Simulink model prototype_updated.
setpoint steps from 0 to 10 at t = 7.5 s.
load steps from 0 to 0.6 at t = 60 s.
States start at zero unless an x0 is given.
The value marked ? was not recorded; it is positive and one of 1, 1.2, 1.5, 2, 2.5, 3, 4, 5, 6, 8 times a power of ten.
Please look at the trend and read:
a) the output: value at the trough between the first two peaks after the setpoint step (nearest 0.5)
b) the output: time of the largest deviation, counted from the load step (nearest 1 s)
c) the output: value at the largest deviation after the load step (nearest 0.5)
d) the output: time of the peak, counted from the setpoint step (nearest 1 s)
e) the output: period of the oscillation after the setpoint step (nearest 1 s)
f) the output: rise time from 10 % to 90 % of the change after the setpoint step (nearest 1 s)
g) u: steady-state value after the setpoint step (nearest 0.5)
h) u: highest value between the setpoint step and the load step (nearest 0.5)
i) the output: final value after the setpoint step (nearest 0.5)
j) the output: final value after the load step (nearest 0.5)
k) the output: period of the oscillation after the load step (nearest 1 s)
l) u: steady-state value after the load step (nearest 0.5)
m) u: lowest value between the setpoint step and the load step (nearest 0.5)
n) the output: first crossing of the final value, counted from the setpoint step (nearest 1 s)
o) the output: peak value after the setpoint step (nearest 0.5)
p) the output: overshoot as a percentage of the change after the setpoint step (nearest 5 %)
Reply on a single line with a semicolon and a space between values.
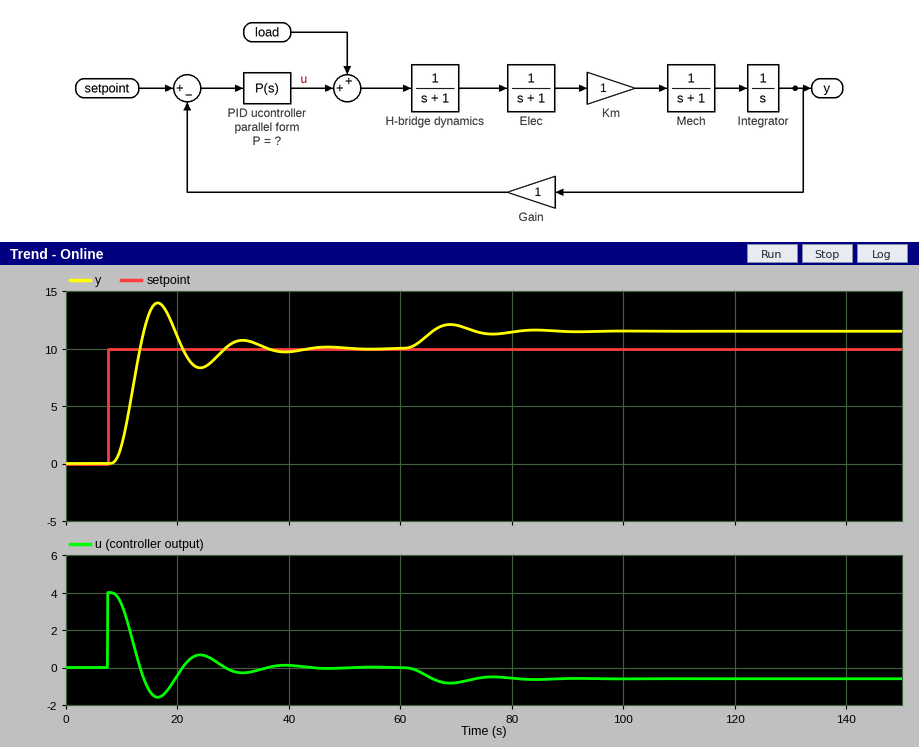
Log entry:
8.5; 9 s; 12.0; 9 s; 15 s; 3 s; 0.0; 4.0; 10.0; 11.5; 15 s; -0.5; -1.5; 6 s; 14.0; 40 %
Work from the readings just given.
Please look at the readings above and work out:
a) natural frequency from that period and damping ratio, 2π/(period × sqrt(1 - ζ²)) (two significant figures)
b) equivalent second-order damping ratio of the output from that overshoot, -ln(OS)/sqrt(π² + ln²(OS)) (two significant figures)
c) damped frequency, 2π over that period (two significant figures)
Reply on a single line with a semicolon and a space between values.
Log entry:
0.44 rad/s; 0.28; 0.42 rad/s
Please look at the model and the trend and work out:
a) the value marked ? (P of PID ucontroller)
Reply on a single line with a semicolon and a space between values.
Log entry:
0.4
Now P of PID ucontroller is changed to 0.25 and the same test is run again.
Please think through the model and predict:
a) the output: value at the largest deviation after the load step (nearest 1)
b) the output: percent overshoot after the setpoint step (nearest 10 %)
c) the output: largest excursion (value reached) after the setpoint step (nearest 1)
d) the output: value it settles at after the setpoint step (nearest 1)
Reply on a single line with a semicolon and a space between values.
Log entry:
13; 20 %; 12; 10
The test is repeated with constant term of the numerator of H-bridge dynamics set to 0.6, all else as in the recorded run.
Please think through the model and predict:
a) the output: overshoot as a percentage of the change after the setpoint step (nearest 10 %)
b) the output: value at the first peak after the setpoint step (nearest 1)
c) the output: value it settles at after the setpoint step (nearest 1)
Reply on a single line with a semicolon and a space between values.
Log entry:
20 %; 12; 10
